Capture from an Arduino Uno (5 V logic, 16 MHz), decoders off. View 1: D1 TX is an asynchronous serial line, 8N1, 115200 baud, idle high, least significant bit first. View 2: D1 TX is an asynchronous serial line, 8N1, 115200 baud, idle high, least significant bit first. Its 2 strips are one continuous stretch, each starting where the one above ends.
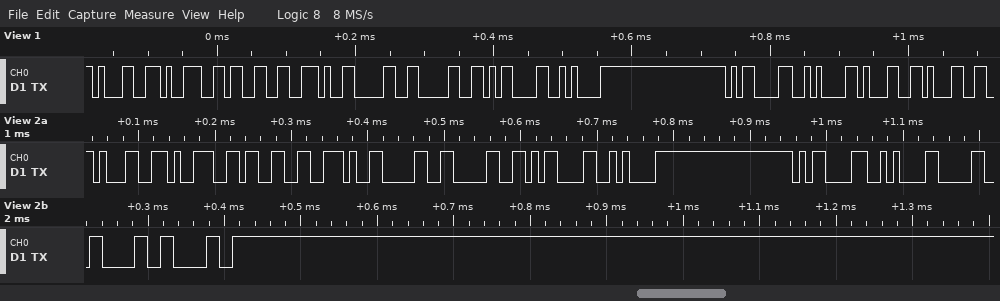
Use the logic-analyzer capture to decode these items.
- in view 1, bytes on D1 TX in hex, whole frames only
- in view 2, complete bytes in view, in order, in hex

31 39 33 2E 30 30 0D 0A 0D 0A 31 31
31 39 33 2E 30 30 0D 0A 0D 0A 30 30 30
